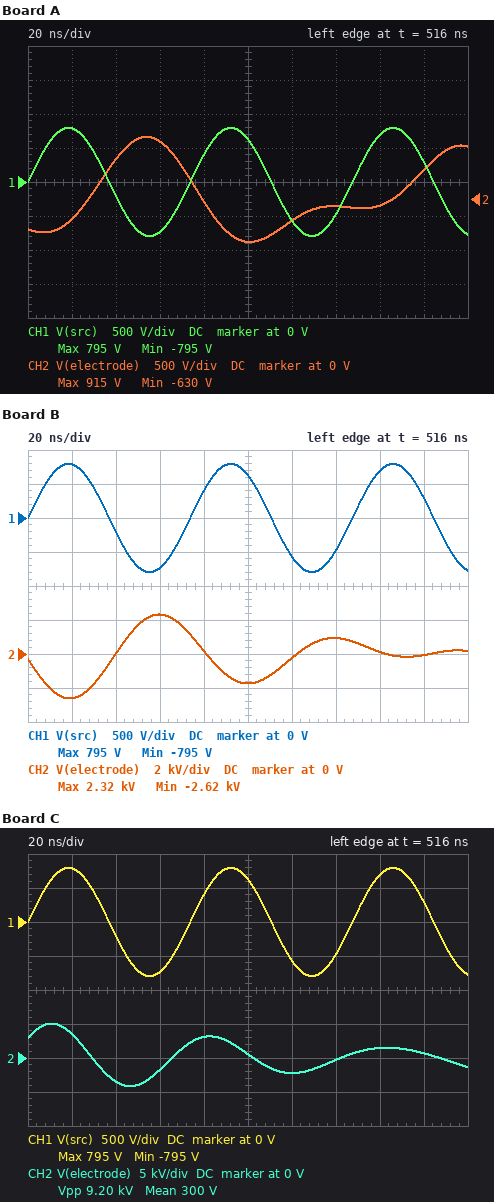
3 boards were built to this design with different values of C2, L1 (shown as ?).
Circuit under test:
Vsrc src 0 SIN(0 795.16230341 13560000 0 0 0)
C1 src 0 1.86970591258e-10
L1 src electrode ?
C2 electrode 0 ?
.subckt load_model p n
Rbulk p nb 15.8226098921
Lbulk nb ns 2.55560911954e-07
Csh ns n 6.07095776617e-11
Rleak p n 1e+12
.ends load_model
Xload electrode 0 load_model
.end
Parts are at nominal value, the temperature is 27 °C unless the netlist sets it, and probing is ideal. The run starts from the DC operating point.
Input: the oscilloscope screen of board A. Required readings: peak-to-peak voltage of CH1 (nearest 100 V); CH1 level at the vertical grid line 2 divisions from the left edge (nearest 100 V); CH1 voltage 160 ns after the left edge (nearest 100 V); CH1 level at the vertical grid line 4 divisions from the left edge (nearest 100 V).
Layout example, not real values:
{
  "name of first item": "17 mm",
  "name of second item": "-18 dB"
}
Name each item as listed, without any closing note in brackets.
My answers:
{
  "peak-to-peak voltage of CH1": "1.6 kV",
  "CH1 level at the vertical grid line 2 divisions from the left edge": "-200 V",
  "CH1 voltage 160 ns after the left edge": "700 V",
  "CH1 level at the vertical grid line 4 divisions from the left edge": "400 V"
}
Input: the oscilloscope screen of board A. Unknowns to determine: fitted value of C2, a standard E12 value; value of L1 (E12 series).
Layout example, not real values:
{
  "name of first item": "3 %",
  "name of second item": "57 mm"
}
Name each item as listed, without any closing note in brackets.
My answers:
{
  "fitted value of C2, a standard E12 value": "390 pF",
  "value of L1": "1 µH"
}
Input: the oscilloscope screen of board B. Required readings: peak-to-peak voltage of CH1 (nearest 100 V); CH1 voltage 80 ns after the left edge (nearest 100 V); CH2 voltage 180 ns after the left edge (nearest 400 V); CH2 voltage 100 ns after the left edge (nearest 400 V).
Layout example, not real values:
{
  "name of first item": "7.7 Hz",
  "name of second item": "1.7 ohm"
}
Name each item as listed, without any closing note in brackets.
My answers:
{
  "peak-to-peak voltage of CH1": "1.6 kV",
  "CH1 voltage 80 ns after the left edge": "400 V",
  "CH2 voltage 180 ns after the left edge": "0 V",
  "CH2 voltage 100 ns after the left edge": "-1.6 kV"
}
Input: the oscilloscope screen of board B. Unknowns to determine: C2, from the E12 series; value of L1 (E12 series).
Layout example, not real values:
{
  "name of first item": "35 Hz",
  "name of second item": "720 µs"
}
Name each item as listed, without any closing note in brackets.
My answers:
{
  "C2, from the E12 series": "330 pF",
  "value of L1": "560 nH"
}
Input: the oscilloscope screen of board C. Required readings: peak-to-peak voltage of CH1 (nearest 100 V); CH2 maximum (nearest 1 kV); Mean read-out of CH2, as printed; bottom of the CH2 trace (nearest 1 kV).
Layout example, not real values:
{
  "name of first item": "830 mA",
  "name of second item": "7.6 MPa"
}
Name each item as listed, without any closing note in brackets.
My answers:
{
  "peak-to-peak voltage of CH1": "1.6 kV",
  "CH2 maximum": "5 kV",
  "Mean read-out of CH2, as printed": "300 V",
  "bottom of the CH2 trace": "-4 kV"
}
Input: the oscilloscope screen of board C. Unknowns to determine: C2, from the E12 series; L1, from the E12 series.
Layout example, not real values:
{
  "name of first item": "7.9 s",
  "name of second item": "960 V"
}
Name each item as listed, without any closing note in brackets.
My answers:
{
  "C2, from the E12 series": "680 pF",
  "L1, from the E12 series": "150 nH"
}
